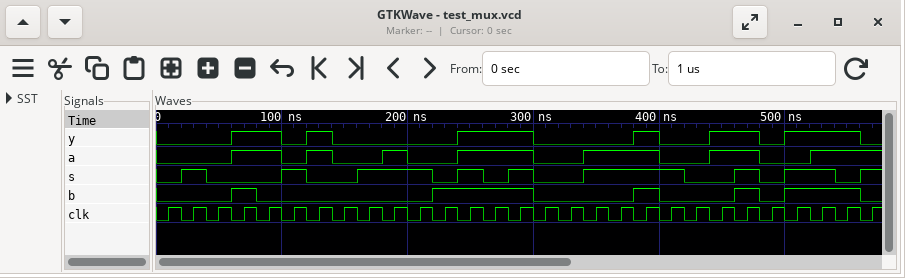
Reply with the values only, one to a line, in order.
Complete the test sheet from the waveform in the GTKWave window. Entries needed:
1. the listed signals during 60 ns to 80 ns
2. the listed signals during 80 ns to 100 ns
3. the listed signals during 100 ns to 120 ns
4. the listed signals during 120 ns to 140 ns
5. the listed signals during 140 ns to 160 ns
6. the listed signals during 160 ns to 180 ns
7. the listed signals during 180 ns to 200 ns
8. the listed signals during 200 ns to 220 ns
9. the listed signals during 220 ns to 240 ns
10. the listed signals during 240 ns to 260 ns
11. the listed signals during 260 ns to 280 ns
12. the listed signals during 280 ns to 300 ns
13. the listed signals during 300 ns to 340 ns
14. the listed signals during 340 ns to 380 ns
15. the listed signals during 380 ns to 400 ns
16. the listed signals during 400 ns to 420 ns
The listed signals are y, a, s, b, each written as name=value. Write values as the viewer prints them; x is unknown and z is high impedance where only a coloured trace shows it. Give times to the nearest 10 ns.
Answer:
y=1, a=1, s=0, b=1
y=1, a=1, s=0, b=0
y=0, a=0, s=1, b=0
y=1, a=1, s=0, b=0
y=0, a=0, s=0, b=0
y=0, a=0, s=1, b=0
y=0, a=1, s=1, b=0
y=0, a=0, s=1, b=0
y=0, a=0, s=0, b=1
y=1, a=1, s=1, b=1
y=1, a=1, s=0, b=1
y=1, a=1, s=1, b=1
y=0, a=0, s=0, b=0
y=0, a=1, s=1, b=0
y=1, a=1, s=1, b=1
y=0, a=0, s=1, b=0
